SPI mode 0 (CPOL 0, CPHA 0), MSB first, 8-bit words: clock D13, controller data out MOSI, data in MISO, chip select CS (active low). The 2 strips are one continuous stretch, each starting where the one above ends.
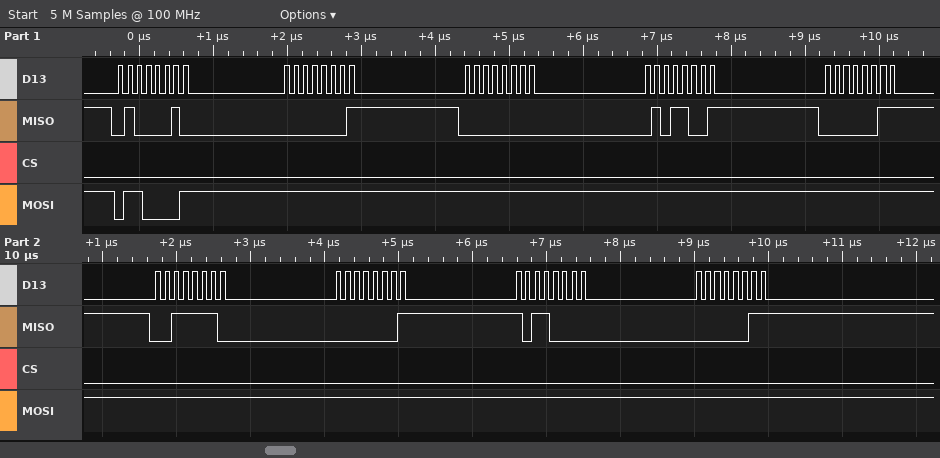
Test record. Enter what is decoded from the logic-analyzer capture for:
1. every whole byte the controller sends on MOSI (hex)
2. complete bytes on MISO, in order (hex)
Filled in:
0x61 0xFF 0xFF 0xFF 0xFF 0xFF 0xFF 0xFF 0xFF
0x42 0x01 0x00 0x59 0x03 0x3E 0x01 0xB0 0x03
